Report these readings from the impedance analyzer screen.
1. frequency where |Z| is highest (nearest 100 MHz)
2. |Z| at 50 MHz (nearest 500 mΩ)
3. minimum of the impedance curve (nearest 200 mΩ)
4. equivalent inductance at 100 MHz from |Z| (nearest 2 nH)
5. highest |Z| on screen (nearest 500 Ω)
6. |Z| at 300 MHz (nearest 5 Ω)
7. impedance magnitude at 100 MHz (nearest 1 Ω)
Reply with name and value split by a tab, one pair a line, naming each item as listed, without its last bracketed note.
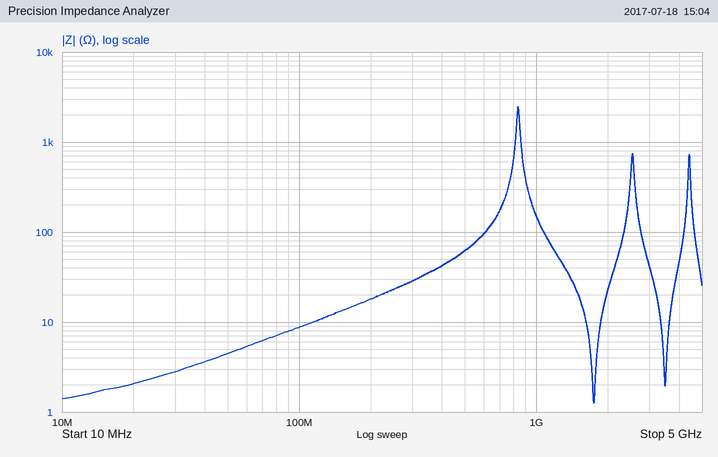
frequency where |Z| is highest	800 MHz
|Z| at 50 MHz	4.5 Ω
minimum of the impedance curve	1.2 Ω
equivalent inductance at 100 MHz from |Z|	14 nH
highest |Z| on screen	2.5 kΩ
|Z| at 300 MHz	30 Ω
impedance magnitude at 100 MHz	9 Ω
